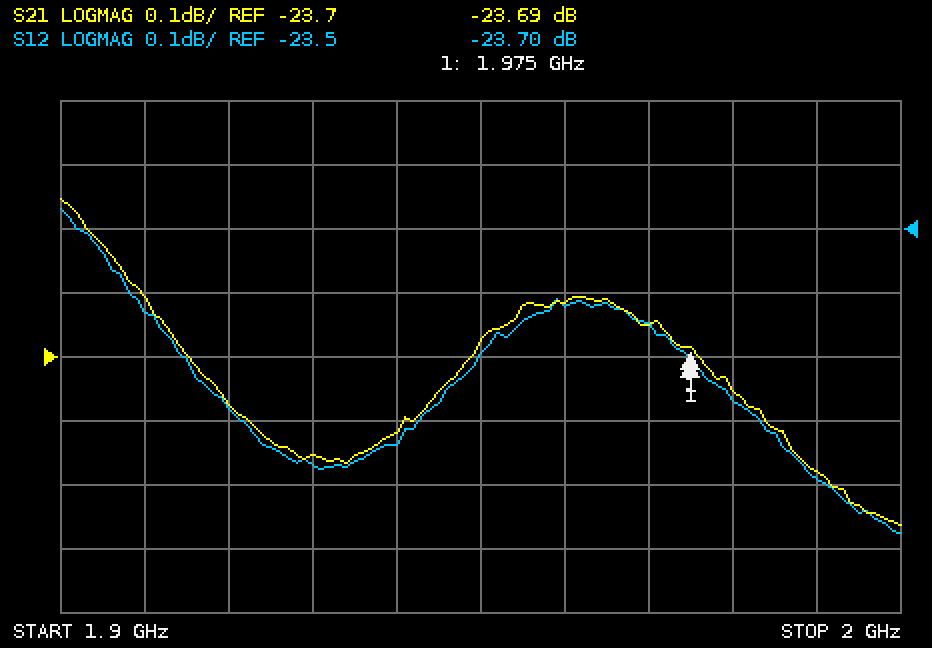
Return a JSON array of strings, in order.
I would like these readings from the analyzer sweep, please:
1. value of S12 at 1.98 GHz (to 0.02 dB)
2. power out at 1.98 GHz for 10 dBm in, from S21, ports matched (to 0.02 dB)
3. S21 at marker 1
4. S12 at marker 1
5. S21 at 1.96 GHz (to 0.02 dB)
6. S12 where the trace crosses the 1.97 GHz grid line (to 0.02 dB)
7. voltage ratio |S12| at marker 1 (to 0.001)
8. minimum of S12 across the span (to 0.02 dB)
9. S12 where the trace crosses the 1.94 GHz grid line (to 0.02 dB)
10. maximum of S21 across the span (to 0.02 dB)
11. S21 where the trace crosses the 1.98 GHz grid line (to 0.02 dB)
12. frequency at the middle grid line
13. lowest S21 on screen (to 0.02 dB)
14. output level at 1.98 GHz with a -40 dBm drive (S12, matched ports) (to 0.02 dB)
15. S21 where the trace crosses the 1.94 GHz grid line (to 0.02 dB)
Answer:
["-23.76 dB", "-13.76 dBm", "-23.69 dB", "-23.70 dB", "-23.62 dB", "-23.64 dB", "0.065", "-23.98 dB", "-23.84 dB", "-23.46 dB", "-23.76 dB", "1.95 GHz", "-23.96 dB", "-63.76 dBm", "-23.82 dB"]
